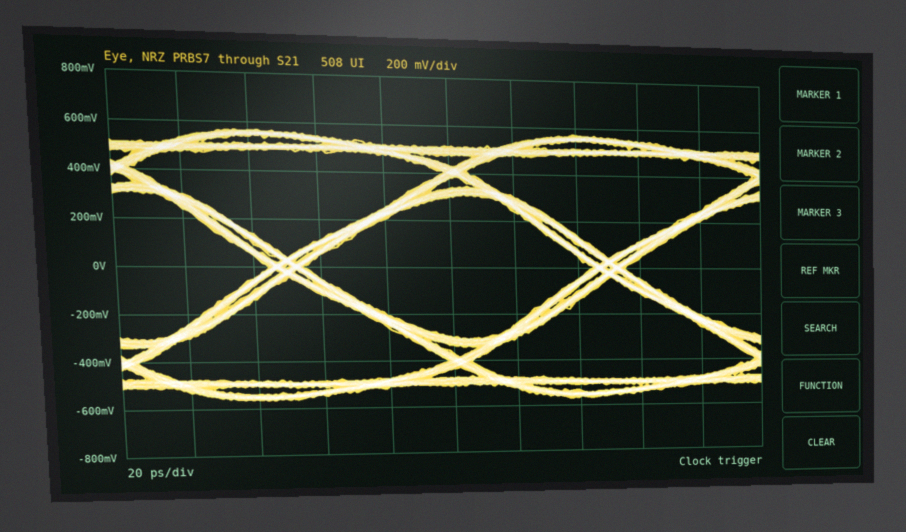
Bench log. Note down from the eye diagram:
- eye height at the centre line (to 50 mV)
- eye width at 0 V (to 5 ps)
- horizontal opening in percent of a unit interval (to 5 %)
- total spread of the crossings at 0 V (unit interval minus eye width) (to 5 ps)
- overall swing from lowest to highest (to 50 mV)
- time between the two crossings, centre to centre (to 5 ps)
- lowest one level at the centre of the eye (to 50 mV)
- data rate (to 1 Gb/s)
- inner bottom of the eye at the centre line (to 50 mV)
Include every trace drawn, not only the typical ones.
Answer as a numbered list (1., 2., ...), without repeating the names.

1. 600 mV
2. 90 ps
3. 90 %
4. 10 ps
5. 1.15 V
6. 100 ps
7. 300 mV
8. 10 Gb/s
9. -300 mV
